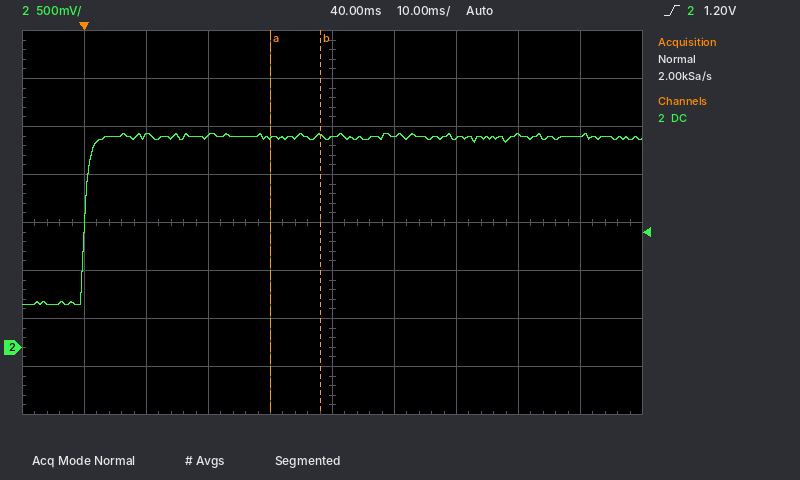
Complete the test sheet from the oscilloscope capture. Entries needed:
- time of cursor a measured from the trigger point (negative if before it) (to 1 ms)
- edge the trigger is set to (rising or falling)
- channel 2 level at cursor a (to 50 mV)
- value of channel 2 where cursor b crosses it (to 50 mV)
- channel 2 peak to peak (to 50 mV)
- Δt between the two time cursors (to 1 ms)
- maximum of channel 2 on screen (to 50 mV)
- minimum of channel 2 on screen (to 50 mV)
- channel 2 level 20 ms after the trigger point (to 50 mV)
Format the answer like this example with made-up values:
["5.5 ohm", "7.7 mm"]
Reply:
["+30 ms", "rising", "2.20 V", "2.20 V", "1.80 V", "8 ms", "2.25 V", "450 mV", "2.20 V"]
